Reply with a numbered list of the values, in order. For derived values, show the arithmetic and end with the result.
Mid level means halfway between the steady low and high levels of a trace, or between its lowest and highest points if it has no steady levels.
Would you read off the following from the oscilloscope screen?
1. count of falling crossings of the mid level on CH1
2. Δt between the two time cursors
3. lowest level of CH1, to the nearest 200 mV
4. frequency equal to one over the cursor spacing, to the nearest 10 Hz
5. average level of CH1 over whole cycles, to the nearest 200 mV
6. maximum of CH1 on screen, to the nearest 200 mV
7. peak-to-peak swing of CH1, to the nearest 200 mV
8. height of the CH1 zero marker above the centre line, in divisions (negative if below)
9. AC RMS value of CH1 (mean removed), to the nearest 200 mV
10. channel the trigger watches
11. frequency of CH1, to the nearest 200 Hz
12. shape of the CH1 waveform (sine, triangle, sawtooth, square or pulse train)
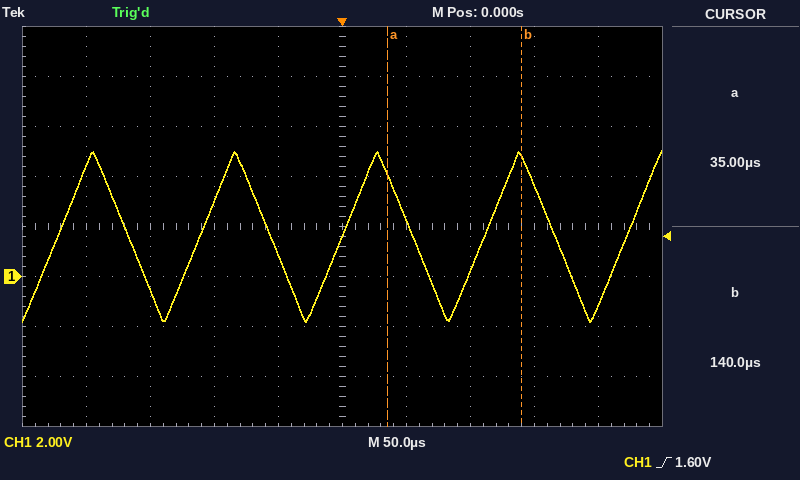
1. 4
2. 140 µs − (35 µs) = 105 µs
3. -1.8 V
4. 1 / 105 µs ≈ 9.52 kHz
5. (5.0 V + (-1.8 V)) / 2 ≈ 1.6 V
6. 5.0 V
7. 5.0 V − (-1.8 V) = 6.8 V
8. -1.0 div
9. 6.8 V / (2√3) ≈ 2.0 V
10. CH1
11. 9.0 kHz
12. triangle
